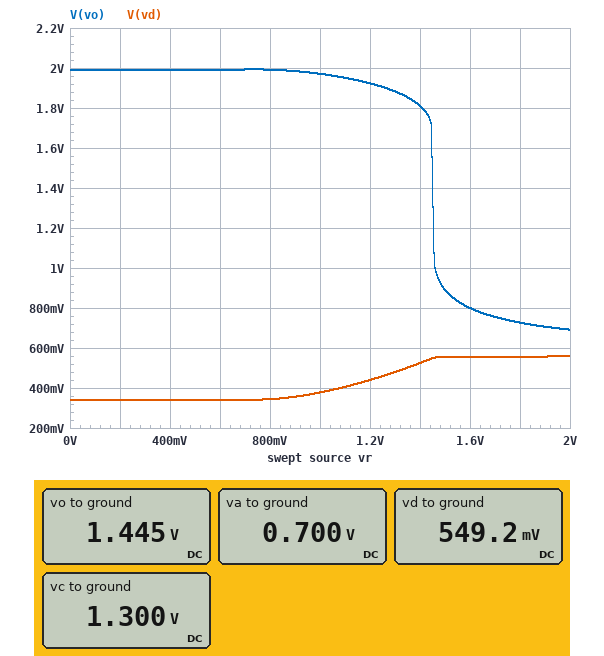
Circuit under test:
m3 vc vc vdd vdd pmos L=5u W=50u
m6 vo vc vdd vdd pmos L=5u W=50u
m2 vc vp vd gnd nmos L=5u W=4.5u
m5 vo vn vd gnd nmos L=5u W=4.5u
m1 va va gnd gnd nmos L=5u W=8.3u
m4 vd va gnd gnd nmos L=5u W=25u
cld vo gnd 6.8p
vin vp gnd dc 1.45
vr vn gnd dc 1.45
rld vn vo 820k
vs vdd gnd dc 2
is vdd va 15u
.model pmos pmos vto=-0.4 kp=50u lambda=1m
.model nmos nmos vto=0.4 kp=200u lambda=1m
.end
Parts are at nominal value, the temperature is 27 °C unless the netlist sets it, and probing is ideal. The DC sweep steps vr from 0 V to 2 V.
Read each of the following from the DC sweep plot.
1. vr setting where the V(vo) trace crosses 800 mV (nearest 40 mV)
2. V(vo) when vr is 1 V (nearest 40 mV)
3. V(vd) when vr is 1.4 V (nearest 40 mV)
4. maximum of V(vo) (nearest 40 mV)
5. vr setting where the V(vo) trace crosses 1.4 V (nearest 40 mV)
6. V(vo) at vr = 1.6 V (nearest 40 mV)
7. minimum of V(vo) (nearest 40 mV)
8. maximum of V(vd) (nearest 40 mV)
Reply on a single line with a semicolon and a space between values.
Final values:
1.60 V; 1.96 V; 520 mV; 2.00 V; 1.44 V; 800 mV; 680 mV; 560 mV
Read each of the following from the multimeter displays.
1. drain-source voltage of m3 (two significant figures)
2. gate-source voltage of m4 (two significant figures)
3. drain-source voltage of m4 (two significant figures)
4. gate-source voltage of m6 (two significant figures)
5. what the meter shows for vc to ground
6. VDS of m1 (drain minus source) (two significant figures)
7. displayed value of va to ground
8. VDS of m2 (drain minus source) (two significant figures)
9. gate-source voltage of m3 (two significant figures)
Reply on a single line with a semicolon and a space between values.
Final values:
-700 mV; 700 mV; 550 mV; -700 mV; 1.300 V; 700 mV; 0.700 V; 750 mV; -700 mV
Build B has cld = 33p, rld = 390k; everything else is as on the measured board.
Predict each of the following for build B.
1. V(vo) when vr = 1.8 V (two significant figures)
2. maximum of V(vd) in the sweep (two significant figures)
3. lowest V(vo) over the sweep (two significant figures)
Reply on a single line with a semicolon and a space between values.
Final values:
740 mV; 570 mV; 710 mV
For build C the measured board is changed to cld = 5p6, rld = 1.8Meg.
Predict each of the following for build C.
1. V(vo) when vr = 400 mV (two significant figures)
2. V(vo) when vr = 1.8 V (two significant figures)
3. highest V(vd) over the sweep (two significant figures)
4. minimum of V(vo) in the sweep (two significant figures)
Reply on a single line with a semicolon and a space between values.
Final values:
2.0 V; 720 mV; 550 mV; 680 mV
